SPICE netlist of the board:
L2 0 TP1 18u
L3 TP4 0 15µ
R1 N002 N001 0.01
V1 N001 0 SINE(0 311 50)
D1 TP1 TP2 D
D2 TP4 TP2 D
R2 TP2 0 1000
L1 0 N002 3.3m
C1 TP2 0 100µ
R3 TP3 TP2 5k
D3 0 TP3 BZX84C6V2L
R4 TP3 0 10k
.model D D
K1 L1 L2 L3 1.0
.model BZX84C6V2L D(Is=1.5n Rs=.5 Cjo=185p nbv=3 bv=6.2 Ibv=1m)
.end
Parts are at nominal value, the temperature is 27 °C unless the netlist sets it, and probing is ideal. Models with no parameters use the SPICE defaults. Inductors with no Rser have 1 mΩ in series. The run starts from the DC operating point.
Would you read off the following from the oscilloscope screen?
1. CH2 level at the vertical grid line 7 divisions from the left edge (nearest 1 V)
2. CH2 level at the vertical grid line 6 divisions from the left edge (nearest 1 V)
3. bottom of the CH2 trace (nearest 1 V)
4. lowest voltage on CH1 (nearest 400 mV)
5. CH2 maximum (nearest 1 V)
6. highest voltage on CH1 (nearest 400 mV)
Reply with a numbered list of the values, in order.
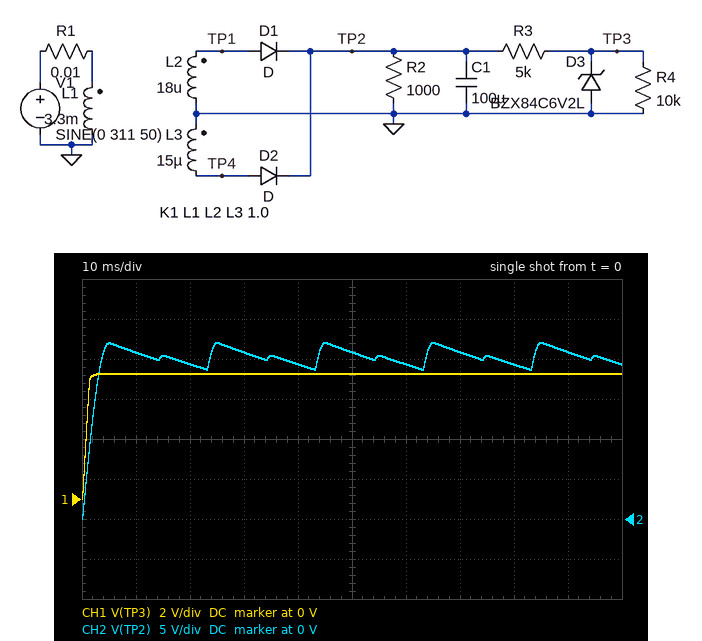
1. 21 V
2. 19 V
3. 0 V
4. 0 V
5. 22 V
6. 6.4 V
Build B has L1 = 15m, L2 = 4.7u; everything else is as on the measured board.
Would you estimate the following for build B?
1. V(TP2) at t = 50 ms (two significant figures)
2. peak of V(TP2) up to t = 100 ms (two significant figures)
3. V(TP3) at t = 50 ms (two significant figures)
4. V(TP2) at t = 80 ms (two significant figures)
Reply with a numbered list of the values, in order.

1. 7.8 V
2. 9.1 V
3. 5.2 V
4. 8.7 V
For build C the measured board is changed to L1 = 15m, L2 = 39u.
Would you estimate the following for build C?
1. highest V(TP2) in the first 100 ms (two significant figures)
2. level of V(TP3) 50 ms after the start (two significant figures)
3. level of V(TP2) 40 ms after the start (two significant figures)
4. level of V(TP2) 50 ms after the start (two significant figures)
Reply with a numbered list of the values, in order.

1. 15 V
2. 6.2 V
3. 13 V
4. 14 V
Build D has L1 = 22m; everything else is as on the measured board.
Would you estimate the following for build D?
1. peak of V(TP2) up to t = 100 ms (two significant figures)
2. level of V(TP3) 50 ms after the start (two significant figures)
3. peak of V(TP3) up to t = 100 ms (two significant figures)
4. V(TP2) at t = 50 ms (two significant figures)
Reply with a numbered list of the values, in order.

1. 8.2 V
2. 5.2 V
3. 5.4 V
4. 7.8 V
